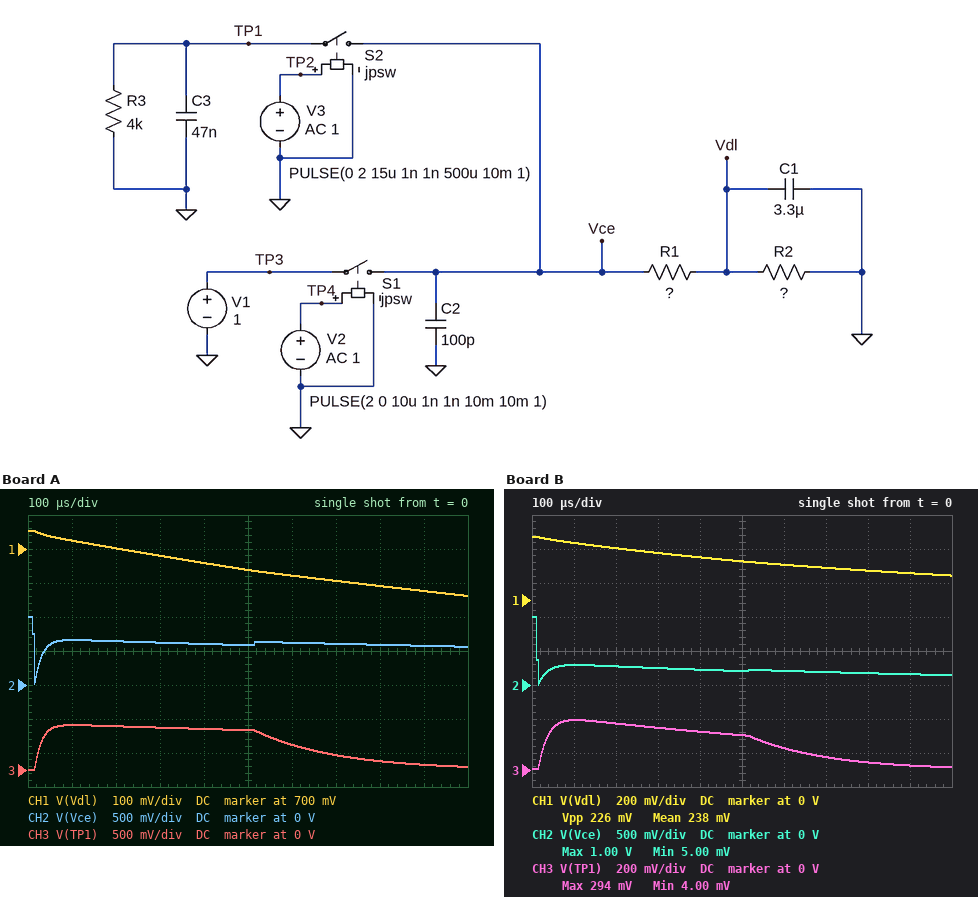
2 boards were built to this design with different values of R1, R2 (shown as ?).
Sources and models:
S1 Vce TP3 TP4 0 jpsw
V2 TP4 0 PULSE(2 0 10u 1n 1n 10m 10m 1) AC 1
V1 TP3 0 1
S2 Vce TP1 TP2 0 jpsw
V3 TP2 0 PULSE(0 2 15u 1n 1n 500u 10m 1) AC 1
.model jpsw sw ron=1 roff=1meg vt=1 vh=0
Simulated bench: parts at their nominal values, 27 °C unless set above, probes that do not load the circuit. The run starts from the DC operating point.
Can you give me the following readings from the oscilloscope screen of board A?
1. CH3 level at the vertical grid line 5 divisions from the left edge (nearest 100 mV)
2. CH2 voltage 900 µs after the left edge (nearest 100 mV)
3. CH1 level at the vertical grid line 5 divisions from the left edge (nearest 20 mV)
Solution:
600 mV
600 mV
640 mV
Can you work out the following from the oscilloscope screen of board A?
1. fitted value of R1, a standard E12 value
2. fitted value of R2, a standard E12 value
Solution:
390 Ω
1.2 kΩ
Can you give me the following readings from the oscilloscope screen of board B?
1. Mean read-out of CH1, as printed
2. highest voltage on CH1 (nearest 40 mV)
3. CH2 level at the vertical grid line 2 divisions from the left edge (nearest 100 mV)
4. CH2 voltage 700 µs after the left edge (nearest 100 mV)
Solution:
238 mV
360 mV
300 mV
200 mV
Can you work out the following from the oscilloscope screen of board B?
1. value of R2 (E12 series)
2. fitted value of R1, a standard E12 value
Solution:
330 Ω
560 Ω
